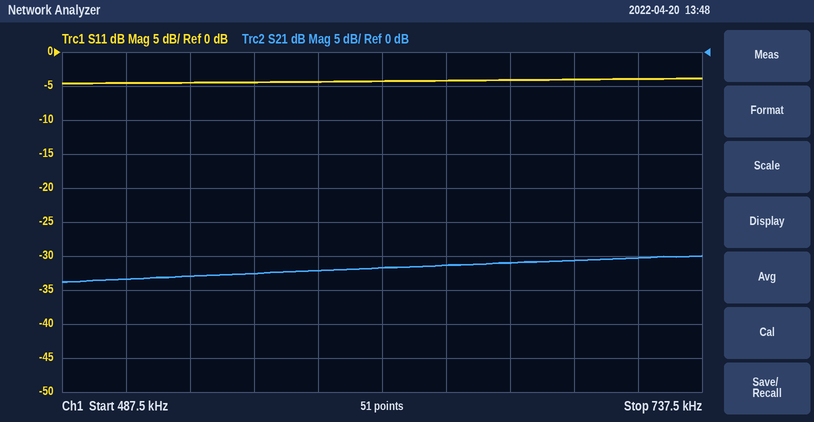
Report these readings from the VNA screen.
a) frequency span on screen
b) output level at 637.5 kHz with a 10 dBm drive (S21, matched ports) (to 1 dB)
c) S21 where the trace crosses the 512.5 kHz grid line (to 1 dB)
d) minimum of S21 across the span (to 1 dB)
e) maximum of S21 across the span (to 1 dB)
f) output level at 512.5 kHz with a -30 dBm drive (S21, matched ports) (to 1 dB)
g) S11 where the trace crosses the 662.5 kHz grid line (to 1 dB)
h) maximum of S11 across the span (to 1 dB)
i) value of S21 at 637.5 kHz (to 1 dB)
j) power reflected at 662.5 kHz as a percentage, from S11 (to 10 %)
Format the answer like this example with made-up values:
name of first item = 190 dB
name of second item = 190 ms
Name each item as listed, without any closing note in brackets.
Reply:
frequency span on screen = 250 kHz
output level at 637.5 kHz with a 10 dBm drive (S21, matched ports) = -21 dBm
S21 where the trace crosses the 512.5 kHz grid line = -33 dB
minimum of S21 across the span = -34 dB
maximum of S21 across the span = -30 dB
output level at 512.5 kHz with a -30 dBm drive (S21, matched ports) = -63 dBm
S11 where the trace crosses the 662.5 kHz grid line = -4 dB
maximum of S11 across the span = -4 dB
value of S21 at 637.5 kHz = -31 dB
power reflected at 662.5 kHz as a percentage, from S11 = 40 %
